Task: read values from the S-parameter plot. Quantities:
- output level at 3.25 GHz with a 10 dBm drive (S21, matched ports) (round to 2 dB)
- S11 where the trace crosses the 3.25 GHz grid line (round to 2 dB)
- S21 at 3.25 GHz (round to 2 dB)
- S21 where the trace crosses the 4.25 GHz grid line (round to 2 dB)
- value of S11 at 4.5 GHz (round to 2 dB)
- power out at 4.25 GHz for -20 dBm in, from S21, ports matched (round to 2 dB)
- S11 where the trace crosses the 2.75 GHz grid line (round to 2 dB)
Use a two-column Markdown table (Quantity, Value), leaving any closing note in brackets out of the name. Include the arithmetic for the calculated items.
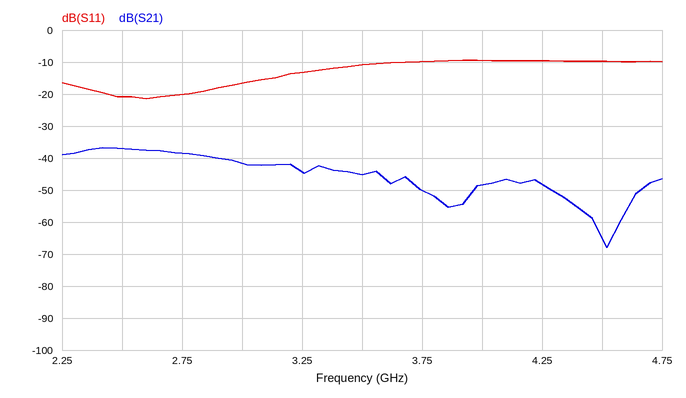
| Quantity | Value |
|---|---|
| output level at 3.25 GHz with a 10 dBm drive (S21, matched ports) | 10 dBm + (-44 dB) = -34 dBm |
| S11 where the trace crosses the 3.25 GHz grid line | -14 dB |
| S21 at 3.25 GHz | -44 dB |
| S21 where the trace crosses the 4.25 GHz grid line | -48 dB |
| value of S11 at 4.5 GHz | -10 dB |
| power out at 4.25 GHz for -20 dBm in, from S21, ports matched | -20 dBm + (-48 dB) = -68 dBm |
| S11 where the trace crosses the 2.75 GHz grid line | -20 dB |
